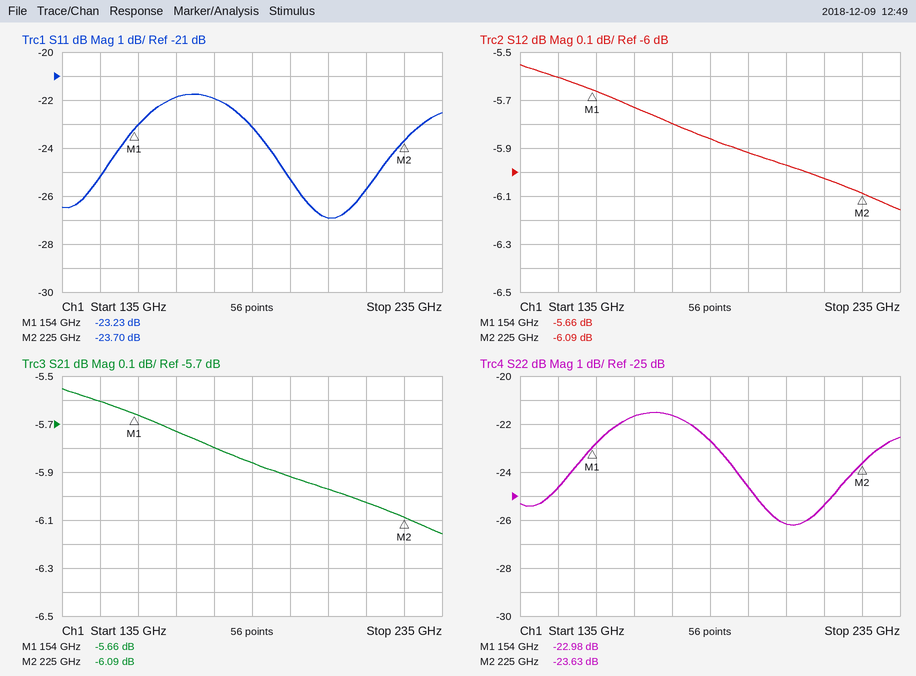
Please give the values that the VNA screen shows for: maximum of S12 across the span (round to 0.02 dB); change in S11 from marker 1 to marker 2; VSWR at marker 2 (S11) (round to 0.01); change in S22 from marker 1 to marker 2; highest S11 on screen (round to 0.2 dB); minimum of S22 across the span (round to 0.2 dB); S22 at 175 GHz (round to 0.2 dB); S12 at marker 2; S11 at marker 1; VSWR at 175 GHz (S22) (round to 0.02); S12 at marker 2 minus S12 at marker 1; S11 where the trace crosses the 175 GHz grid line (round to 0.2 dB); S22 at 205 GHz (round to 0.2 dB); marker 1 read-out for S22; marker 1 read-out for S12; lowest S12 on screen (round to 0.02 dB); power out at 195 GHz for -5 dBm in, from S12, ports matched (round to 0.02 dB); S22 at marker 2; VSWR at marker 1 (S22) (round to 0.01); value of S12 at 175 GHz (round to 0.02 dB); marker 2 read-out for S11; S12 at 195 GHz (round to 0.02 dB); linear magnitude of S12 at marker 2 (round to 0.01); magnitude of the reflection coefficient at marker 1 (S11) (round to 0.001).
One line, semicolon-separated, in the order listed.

-5.56 dB; -0.47 dB; 1.14; -0.65 dB; -21.8 dB; -26.2 dB; -21.6 dB; -6.09 dB; -23.23 dB; 1.18; -0.43 dB; -22.0 dB; -26.2 dB; -22.98 dB; -5.66 dB; -6.16 dB; -10.92 dBm; -23.63 dB; 1.15; -5.80 dB; -23.70 dB; -5.92 dB; 0.50; 0.069
